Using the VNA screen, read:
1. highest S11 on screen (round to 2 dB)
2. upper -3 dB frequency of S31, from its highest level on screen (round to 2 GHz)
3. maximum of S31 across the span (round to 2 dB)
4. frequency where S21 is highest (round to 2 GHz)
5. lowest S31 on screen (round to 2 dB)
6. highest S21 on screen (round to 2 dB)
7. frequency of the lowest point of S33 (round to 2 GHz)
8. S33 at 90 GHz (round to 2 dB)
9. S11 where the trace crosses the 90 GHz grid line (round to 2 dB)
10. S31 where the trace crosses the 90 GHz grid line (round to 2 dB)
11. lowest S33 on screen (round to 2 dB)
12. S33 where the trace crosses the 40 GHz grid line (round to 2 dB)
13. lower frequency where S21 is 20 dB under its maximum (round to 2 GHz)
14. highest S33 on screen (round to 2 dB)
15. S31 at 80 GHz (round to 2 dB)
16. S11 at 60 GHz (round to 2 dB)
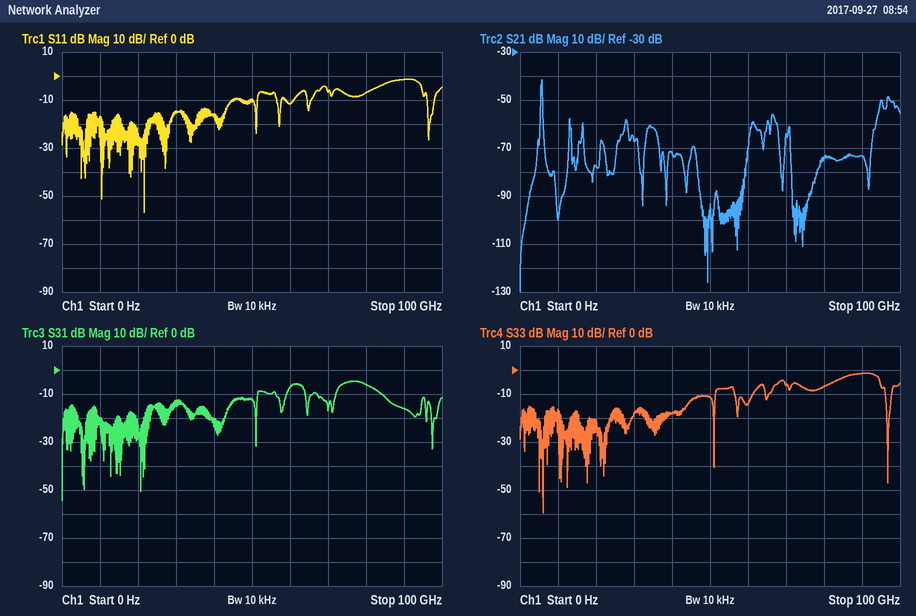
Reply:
-2 dB
82 GHz
-4 dB
6 GHz
-54 dB
-42 dB
6 GHz
-2 dB
-2 dB
-16 dB
-60 dB
-18 dB
6 GHz
-2 dB
-6 dB
-12 dB
